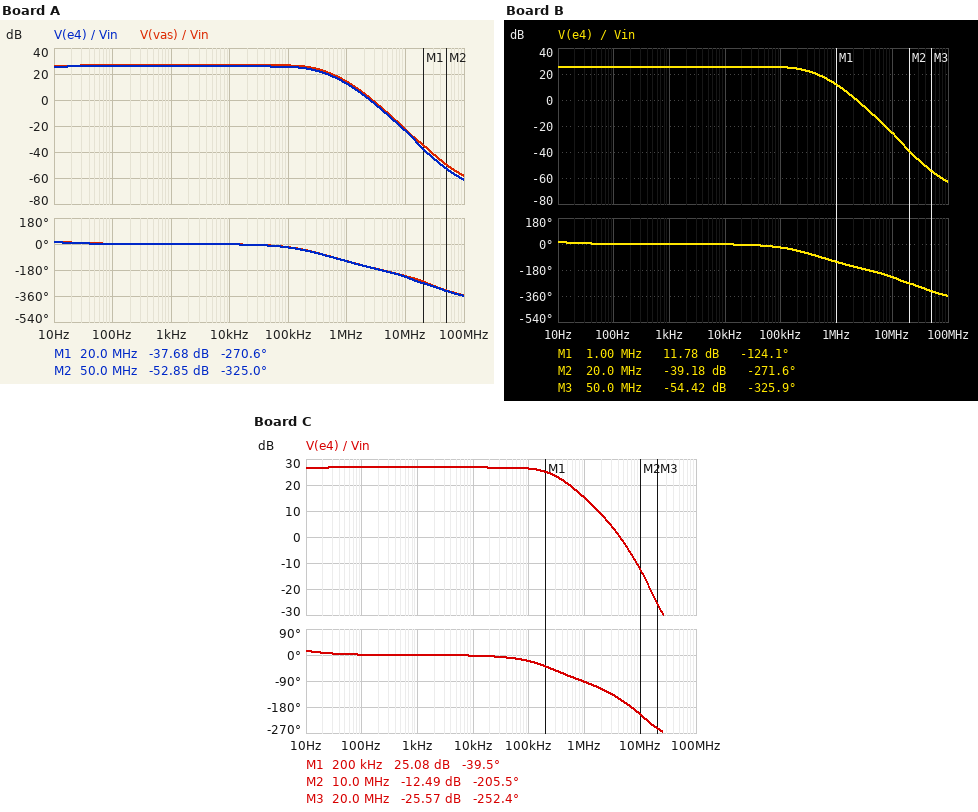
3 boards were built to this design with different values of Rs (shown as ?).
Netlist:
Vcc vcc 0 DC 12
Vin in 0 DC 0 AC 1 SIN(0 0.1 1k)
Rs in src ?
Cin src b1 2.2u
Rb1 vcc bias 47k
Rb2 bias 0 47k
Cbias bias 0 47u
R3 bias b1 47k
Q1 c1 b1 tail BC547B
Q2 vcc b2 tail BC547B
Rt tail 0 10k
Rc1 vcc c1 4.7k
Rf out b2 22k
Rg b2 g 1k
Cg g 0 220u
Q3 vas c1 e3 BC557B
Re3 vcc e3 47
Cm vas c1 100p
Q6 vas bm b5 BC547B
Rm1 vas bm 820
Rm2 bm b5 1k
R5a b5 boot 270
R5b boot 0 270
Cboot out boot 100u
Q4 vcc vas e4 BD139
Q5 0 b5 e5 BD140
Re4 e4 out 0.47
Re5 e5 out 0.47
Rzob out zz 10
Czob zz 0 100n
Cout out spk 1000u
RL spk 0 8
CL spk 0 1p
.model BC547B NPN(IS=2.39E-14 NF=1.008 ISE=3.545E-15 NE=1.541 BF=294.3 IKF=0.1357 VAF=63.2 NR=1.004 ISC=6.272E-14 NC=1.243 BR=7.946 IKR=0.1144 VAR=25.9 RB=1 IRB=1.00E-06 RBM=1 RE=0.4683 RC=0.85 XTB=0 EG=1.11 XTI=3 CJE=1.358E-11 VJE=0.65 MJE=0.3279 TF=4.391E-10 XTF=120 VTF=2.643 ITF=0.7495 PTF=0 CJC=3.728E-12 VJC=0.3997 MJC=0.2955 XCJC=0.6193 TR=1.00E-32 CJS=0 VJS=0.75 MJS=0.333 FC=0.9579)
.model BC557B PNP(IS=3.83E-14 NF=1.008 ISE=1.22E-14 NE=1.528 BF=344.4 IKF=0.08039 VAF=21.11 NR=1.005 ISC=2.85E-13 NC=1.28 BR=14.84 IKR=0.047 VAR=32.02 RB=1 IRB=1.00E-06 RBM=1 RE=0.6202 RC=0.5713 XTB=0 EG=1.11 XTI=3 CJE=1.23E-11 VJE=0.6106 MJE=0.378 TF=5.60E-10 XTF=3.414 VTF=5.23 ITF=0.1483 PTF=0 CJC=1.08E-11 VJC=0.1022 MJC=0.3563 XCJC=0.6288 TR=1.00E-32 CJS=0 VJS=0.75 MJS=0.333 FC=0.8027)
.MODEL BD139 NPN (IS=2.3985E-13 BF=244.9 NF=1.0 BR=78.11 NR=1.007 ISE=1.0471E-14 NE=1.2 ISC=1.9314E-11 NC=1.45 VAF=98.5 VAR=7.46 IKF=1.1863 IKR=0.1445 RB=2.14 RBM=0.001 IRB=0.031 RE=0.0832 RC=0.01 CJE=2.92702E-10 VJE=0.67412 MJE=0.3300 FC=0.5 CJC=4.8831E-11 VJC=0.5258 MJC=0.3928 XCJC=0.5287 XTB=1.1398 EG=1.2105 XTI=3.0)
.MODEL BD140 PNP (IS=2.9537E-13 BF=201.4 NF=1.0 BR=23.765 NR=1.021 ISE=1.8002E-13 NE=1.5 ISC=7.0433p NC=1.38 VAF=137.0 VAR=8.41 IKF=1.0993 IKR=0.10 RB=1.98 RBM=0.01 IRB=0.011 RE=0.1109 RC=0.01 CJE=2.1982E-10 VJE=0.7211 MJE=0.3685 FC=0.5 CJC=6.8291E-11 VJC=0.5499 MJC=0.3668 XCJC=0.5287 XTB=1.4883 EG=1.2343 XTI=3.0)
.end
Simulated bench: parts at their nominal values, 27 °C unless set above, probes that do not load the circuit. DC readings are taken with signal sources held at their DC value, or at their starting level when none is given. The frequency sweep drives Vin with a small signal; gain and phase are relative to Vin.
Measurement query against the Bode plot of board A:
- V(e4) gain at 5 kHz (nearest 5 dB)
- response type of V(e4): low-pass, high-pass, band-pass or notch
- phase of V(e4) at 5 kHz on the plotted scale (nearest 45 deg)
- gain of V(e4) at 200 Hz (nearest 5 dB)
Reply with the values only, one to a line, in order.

25 dB
low-pass
0 deg
25 dB
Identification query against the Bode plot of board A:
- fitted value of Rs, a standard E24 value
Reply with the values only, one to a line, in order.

5.6 kΩ
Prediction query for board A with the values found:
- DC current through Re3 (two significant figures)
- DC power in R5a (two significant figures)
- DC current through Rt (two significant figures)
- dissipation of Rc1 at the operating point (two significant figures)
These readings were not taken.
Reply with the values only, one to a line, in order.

9.8 mA
26 mW
530 µA
280 µW
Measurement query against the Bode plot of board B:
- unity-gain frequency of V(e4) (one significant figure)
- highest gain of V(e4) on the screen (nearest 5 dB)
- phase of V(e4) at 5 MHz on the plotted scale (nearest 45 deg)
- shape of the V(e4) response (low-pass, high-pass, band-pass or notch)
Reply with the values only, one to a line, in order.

2 MHz
25 dB
-180 deg
low-pass
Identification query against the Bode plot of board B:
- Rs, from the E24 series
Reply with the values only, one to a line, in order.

6.8 kΩ
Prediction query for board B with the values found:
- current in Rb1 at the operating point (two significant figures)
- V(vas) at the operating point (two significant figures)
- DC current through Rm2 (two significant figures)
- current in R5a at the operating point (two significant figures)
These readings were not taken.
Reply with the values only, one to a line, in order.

130 µA
6.6 V
700 µA
9.8 mA
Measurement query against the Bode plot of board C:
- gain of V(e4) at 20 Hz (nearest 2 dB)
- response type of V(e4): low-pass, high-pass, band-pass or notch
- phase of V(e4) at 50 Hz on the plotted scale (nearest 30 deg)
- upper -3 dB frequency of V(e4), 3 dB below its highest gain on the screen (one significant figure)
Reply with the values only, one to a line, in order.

26 dB
low-pass
0 deg
300 kHz
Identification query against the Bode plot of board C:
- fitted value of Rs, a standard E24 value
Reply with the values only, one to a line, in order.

750 Ω
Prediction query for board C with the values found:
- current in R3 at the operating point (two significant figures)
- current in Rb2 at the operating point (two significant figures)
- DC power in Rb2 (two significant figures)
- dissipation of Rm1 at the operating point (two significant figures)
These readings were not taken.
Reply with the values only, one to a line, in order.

890 nA
130 µA
760 µW
440 µW
